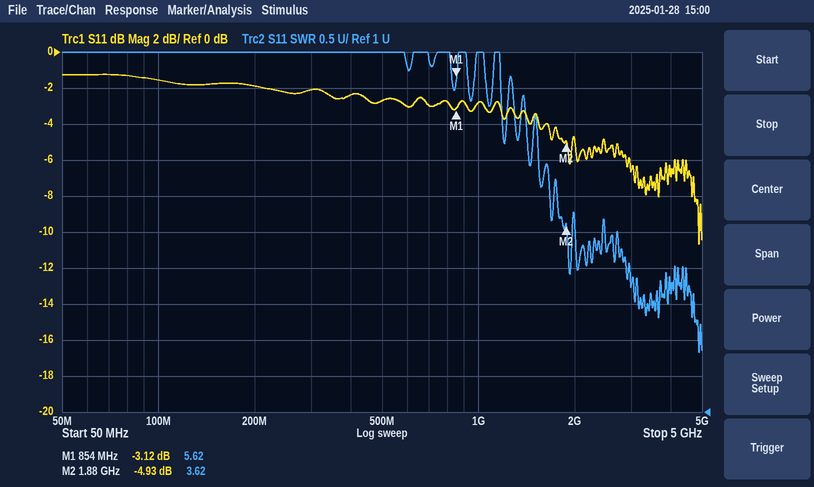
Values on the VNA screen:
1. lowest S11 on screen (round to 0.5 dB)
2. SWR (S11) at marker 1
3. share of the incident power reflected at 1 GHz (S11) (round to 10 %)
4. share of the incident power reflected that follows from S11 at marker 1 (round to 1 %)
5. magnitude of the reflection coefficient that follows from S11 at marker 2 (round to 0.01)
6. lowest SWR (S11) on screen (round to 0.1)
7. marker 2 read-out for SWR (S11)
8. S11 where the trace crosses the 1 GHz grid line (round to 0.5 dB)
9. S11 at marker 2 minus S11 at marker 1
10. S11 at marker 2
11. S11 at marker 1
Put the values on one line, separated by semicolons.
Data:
-10.5 dB; 5.62; 50 %; 49 %; 0.57; 1.8; 3.62; -3.0 dB; -1.81 dB; -4.93 dB; -3.12 dB
